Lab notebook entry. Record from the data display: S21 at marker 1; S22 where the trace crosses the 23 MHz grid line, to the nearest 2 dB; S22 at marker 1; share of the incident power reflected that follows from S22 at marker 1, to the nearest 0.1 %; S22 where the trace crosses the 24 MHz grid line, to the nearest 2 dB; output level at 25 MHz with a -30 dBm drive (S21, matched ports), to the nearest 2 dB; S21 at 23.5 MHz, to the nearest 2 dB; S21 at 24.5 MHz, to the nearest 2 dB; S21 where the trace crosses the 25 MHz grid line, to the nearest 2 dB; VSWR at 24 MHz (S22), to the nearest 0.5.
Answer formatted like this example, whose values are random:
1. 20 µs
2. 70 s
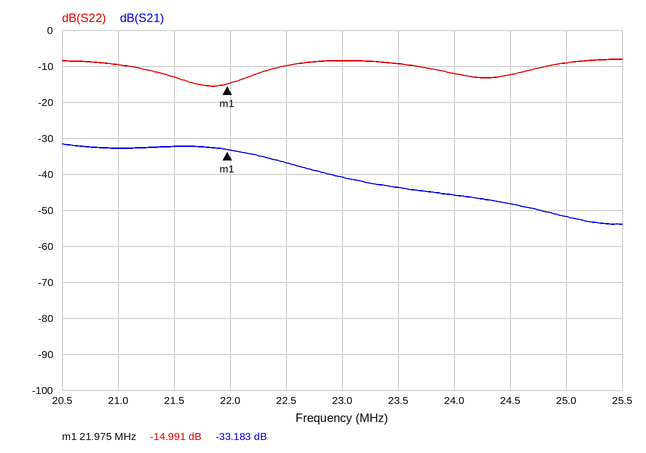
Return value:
1. -33.183 dB
2. -8 dB
3. -14.991 dB
4. 3.2 %
5. -12 dB
6. -82 dBm
7. -44 dB
8. -48 dB
9. -52 dB
10. 1.5
